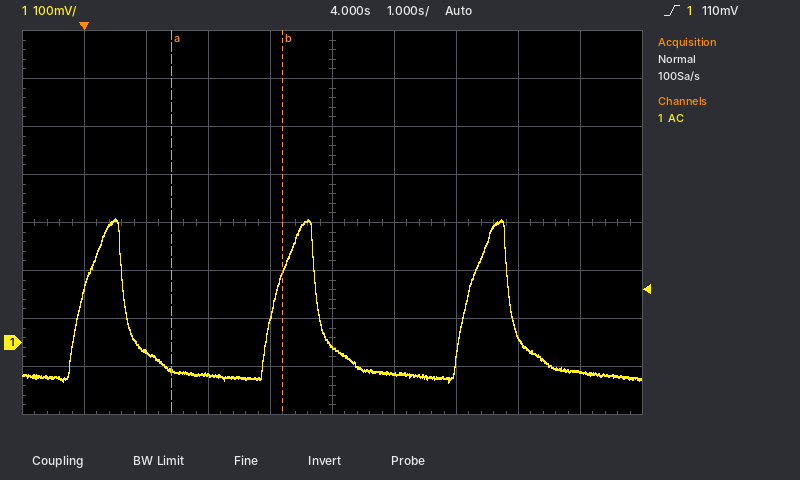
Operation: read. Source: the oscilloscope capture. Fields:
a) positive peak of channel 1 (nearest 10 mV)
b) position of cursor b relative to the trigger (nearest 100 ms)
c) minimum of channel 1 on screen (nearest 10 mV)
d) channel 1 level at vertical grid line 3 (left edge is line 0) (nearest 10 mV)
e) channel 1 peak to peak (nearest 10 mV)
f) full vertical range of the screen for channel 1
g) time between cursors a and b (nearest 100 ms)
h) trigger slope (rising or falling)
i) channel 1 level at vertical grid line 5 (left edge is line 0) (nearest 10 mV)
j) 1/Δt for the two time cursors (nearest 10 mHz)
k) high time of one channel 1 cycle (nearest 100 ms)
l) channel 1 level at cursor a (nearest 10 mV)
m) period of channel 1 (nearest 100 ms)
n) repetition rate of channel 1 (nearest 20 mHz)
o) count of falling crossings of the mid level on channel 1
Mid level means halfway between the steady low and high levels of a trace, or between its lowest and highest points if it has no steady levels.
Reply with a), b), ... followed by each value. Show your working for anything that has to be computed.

a) 260 mV
b) +3.2 s
c) -80 mV
d) -70 mV
e) 260 mV − (-80 mV) = 340 mV
f) 800 mV
g) 1.8 s
h) rising
i) -10 mV
j) 1 / 1.8 s ≈ 560 mHz
k) 700 ms
l) -60 mV
m) 3.1 s
n) 1 / 3.1 s ≈ 323 mHz, so 320 mHz to the nearest 20 mHz
o) 3
